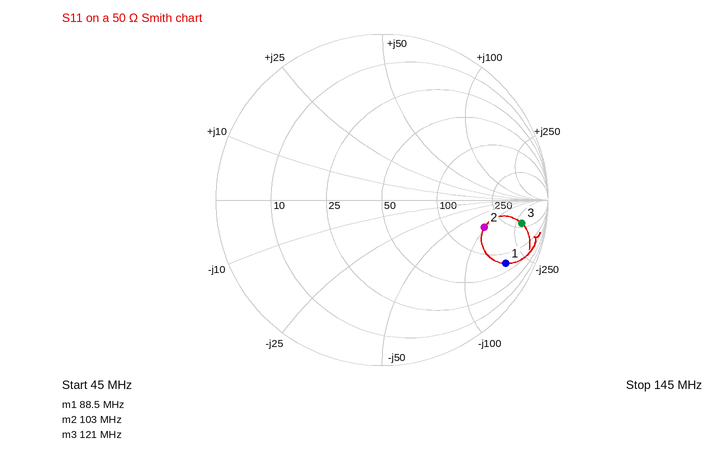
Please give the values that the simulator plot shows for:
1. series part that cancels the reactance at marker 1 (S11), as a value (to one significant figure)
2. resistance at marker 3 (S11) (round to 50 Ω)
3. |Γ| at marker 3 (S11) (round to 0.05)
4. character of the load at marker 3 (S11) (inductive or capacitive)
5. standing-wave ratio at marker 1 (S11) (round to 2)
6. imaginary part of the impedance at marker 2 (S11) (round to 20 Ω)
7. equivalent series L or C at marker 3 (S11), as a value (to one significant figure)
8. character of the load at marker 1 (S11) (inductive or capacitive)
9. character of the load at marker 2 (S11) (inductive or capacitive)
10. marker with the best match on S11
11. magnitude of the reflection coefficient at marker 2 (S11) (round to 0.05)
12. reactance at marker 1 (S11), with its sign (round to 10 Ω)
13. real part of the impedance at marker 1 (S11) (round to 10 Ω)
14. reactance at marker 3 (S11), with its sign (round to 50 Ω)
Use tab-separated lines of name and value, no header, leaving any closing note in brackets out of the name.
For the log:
series part that cancels the reactance at marker 1 (S11), as a value	300 nH
resistance at marker 3 (S11)	300 Ω
|Γ| at marker 3 (S11)	0.85
character of the load at marker 3 (S11)	capacitive
standing-wave ratio at marker 1 (S11)	12
imaginary part of the impedance at marker 2 (S11)	-100 Ω
equivalent series L or C at marker 3 (S11), as a value	4 pF
character of the load at marker 1 (S11)	capacitive
character of the load at marker 2 (S11)	capacitive
marker with the best match on S11	marker 2
magnitude of the reflection coefficient at marker 2 (S11)	0.65
reactance at marker 1 (S11), with its sign	-180 Ω
real part of the impedance at marker 1 (S11)	70 Ω
reactance at marker 3 (S11), with its sign	-300 Ω
